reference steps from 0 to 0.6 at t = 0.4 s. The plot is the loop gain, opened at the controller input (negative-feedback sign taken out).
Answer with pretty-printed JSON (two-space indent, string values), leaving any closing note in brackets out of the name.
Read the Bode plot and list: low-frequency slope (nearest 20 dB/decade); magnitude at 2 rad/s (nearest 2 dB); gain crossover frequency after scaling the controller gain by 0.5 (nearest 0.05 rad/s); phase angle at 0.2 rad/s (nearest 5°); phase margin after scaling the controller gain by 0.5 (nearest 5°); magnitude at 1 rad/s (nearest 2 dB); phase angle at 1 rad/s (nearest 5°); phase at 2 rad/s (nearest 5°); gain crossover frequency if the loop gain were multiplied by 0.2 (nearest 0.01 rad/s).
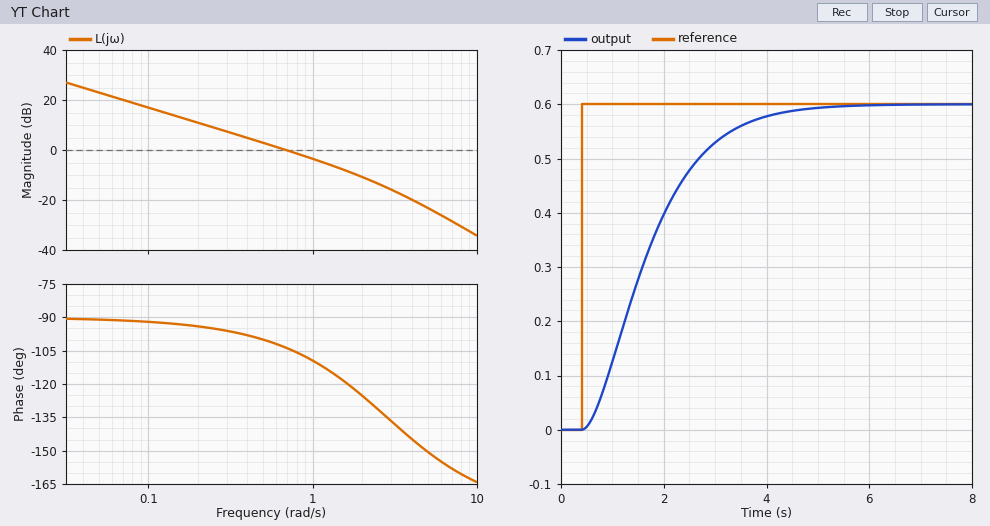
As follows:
{
  "low-frequency slope": "-20 dB/decade",
  "magnitude at 2 rad/s": "-10 dB",
  "gain crossover frequency after scaling the controller gain by 0.5": "0.35 rad/s",
  "phase angle at 0.2 rad/s": "-95°",
  "phase margin after scaling the controller gain by 0.5": "85°",
  "magnitude at 1 rad/s": "-4 dB",
  "phase angle at 1 rad/s": "-110°",
  "phase at 2 rad/s": "-125°",
  "gain crossover frequency if the loop gain were multiplied by 0.2": "0.14 rad/s"
}
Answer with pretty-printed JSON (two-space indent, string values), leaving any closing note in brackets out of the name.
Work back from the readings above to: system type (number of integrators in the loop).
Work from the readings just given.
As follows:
{
  "system type": "1"
}
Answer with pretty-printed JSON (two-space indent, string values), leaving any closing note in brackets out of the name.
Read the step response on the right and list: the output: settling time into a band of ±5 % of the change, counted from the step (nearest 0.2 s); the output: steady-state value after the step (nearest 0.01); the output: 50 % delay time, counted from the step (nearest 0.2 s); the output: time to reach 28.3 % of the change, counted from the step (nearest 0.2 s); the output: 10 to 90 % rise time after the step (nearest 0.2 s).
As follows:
{
  "the output: settling time into a band of ±5 % of the change, counted from the step": "3.4 s",
  "the output: steady-state value after the step": "0.60",
  "the output: 50 % delay time, counted from the step": "1.2 s",
  "the output: time to reach 28.3 % of the change, counted from the step": "0.8 s",
  "the output: 10 to 90 % rise time after the step": "2.4 s"
}
